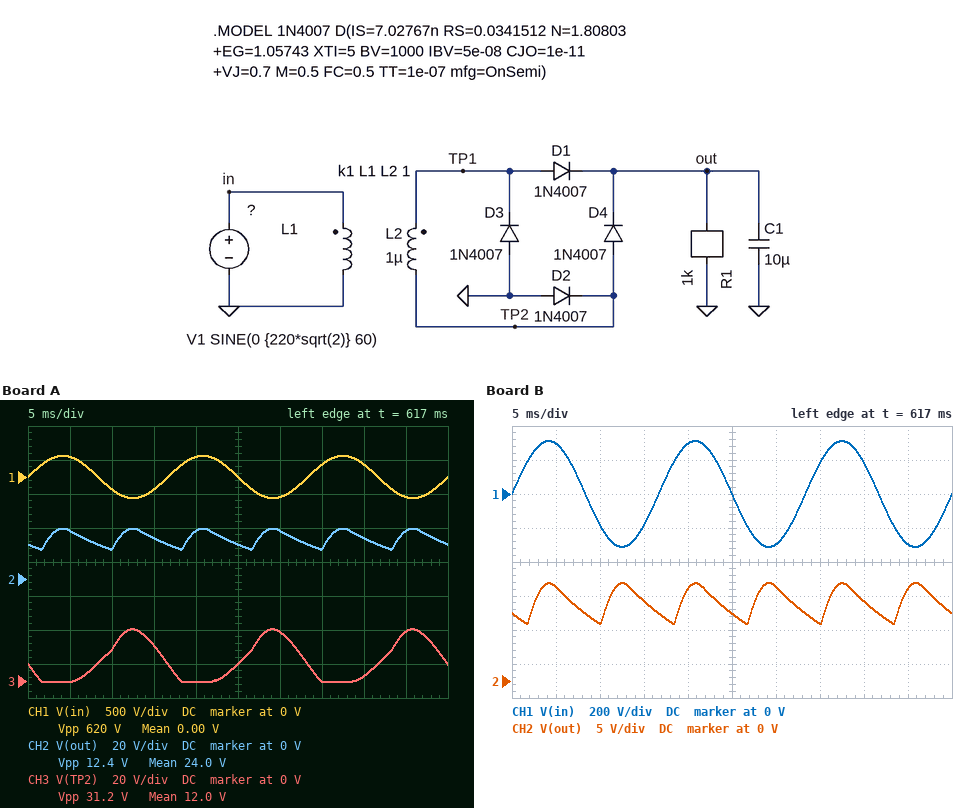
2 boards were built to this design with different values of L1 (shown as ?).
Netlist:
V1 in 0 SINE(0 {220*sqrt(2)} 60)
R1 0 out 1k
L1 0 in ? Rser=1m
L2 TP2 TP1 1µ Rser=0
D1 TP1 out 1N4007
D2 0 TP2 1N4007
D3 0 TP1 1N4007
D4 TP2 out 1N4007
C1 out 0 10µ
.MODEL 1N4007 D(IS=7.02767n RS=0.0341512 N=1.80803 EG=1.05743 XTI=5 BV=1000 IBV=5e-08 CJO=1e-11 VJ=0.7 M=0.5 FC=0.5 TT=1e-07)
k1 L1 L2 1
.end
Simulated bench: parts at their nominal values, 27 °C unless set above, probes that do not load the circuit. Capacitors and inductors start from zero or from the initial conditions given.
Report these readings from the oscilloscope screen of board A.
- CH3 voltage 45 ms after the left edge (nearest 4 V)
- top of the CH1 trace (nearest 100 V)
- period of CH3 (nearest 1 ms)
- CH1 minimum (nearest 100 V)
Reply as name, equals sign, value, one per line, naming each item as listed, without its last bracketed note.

CH3 voltage 45 ms after the left edge = 28 V
top of the CH1 trace = 300 V
period of CH3 = 17 ms
CH1 minimum = -300 V
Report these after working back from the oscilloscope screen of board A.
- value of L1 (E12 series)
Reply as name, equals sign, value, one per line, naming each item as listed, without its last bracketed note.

value of L1 = 100 µH
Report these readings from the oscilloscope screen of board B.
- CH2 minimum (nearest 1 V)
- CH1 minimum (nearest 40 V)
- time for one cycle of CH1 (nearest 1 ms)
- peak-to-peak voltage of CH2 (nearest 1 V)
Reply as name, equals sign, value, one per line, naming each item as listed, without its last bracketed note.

CH2 minimum = 8 V
CH1 minimum = -320 V
time for one cycle of CH1 = 17 ms
peak-to-peak voltage of CH2 = 6 V
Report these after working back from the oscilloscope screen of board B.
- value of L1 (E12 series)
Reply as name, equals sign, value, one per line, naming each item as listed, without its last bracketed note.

value of L1 = 390 µH
